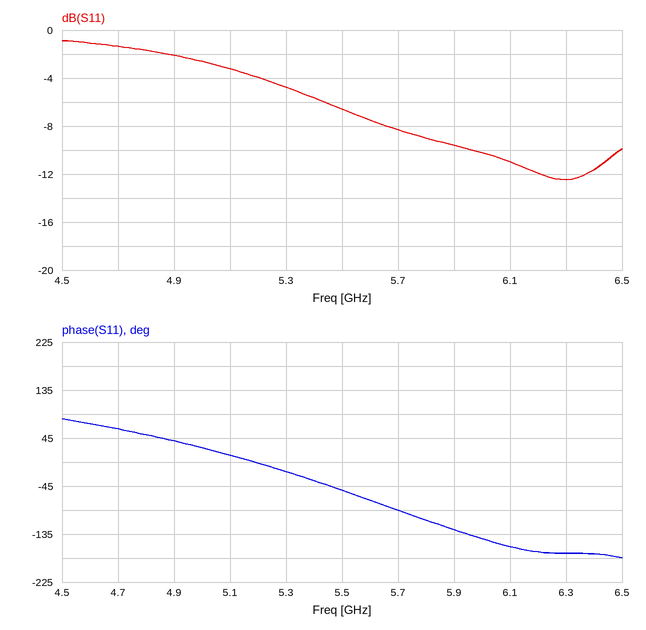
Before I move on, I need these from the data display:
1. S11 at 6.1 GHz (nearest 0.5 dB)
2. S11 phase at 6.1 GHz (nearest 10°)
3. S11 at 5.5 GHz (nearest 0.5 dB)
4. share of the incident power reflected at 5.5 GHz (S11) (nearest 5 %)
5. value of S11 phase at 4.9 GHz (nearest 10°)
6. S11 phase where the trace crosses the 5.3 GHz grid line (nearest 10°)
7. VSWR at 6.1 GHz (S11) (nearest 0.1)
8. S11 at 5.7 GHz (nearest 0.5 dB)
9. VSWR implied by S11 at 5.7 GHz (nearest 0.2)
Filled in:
-11.0 dB
-160°
-6.5 dB
20 %
40°
-20°
1.8
-8.5 dB
2.2
